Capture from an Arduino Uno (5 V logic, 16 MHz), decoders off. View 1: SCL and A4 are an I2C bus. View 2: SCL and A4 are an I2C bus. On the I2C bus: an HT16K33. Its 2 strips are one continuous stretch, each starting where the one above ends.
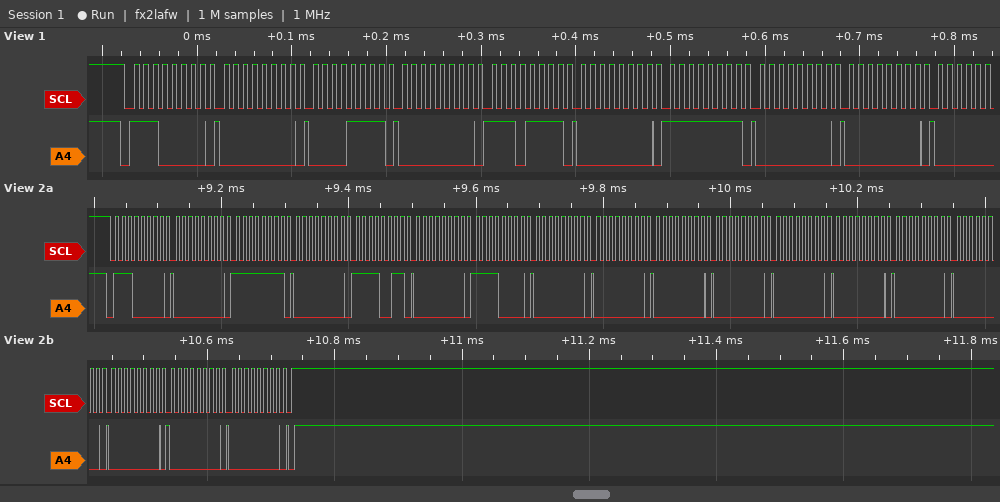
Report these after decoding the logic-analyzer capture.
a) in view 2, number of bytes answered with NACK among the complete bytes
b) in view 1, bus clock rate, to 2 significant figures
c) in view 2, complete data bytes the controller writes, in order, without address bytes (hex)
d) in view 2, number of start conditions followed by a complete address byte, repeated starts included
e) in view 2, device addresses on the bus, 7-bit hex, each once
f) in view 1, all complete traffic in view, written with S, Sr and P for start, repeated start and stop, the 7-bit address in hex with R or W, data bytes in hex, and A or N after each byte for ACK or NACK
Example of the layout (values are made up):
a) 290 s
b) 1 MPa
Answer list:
a) 0
b) 100 kHz
c) 00 FF 00 F3 00 F0 00 00 00 00 00 00 00 00 00 00 00
d) 1
e) 0x70
f) S 70W A 00 A 0F A 00 A EF A 00 A FF A 00 A 00 A
